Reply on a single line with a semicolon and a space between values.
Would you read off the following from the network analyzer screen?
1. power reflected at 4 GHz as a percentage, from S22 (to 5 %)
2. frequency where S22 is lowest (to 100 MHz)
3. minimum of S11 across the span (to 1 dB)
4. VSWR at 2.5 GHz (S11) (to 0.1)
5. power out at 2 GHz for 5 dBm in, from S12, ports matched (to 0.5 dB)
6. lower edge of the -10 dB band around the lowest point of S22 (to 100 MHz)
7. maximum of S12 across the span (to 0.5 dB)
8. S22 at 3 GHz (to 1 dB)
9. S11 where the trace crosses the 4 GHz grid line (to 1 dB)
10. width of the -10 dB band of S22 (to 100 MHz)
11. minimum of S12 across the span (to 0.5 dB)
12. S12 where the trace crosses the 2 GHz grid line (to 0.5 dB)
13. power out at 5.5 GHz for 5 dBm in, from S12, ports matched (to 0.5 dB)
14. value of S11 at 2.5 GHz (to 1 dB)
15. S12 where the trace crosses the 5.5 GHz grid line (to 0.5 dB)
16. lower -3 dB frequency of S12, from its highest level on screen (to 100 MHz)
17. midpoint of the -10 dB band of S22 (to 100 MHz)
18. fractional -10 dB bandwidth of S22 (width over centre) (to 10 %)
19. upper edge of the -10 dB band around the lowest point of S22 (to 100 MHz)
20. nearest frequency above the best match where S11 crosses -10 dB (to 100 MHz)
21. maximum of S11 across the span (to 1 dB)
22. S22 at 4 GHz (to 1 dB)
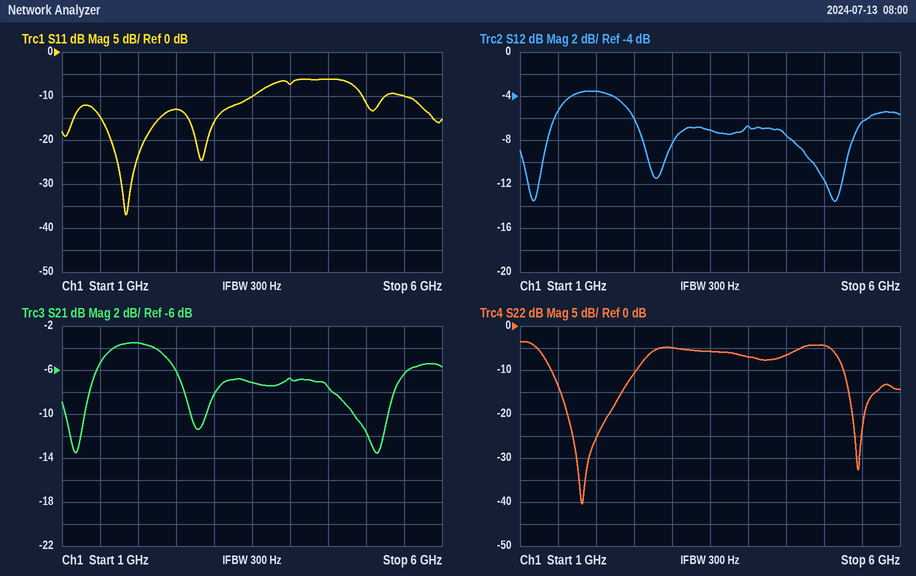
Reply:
20 %; 1.8 GHz; -37 dB; 1.6; 1.5 dBm; 1.4 GHz; -3.5 dB; -5 dB; -7 dB; 1.1 GHz; -13.5 dB; -3.5 dB; -1.5 dBm; -13 dB; -6.5 dB; 1.4 GHz; 2.0 GHz; 60 %; 2.5 GHz; 3.5 GHz; -6 dB; -7 dB
